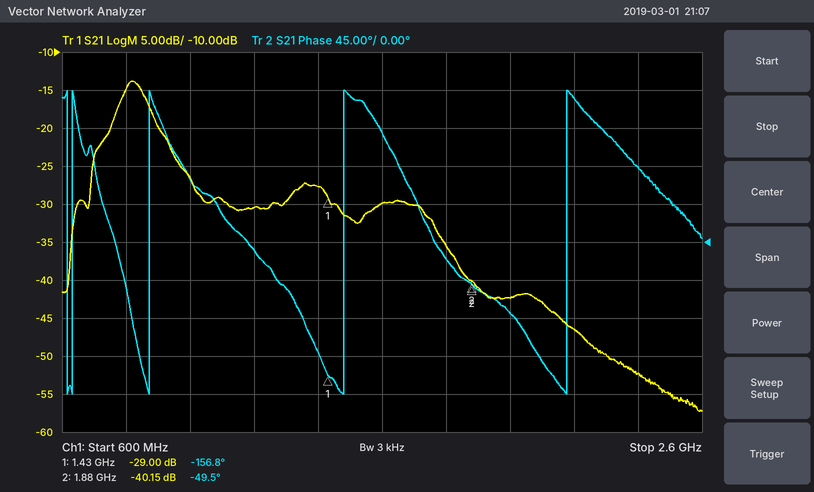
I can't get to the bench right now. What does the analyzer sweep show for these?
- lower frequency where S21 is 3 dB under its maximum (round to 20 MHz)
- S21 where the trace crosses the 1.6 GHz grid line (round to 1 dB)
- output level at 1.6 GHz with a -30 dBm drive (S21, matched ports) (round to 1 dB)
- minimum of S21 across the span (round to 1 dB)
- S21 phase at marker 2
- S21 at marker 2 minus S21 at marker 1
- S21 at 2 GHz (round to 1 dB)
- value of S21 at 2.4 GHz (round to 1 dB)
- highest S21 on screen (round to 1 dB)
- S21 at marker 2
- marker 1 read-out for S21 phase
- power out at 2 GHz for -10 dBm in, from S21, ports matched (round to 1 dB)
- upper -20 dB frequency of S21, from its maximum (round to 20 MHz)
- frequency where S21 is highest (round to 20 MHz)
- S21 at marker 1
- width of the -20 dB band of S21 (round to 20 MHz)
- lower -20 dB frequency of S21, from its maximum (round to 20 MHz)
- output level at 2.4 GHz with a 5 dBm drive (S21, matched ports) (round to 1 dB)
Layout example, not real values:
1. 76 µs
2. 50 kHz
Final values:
1. 780 MHz
2. -30 dB
3. -60 dBm
4. -57 dB
5. -49.5°
6. -11.15 dB
7. -42 dB
8. -52 dB
9. -14 dB
10. -40.15 dB
11. -156.8°
12. -52 dBm
13. 1.78 GHz
14. 820 MHz
15. -29.00 dB
16. 1.14 GHz
17. 640 MHz
18. -47 dBm
